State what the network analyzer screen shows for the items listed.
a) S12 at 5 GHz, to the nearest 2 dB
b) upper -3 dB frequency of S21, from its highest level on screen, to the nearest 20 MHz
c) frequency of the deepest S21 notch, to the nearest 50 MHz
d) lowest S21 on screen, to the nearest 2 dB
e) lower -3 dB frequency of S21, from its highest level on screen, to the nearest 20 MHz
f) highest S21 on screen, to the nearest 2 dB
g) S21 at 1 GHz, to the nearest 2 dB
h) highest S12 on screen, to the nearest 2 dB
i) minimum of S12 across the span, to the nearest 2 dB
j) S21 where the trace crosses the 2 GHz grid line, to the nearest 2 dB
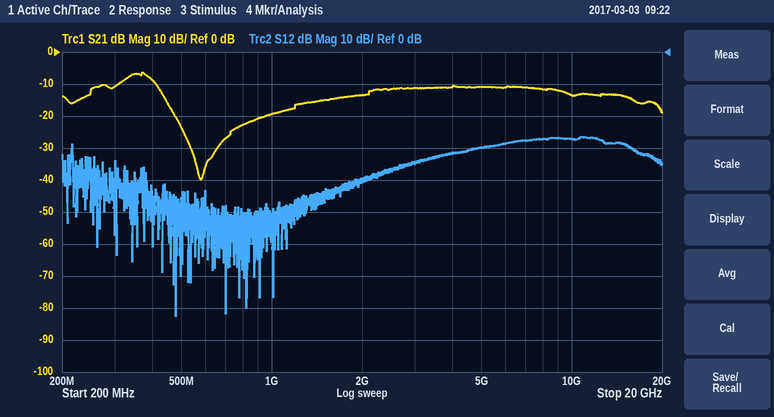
-30 dB
400 MHz
600 MHz
-40 dB
320 MHz
-6 dB
-20 dB
-26 dB
-82 dB
-14 dB
